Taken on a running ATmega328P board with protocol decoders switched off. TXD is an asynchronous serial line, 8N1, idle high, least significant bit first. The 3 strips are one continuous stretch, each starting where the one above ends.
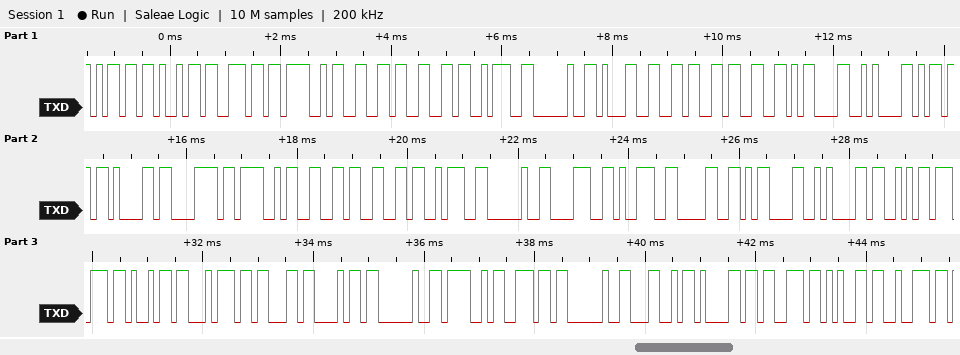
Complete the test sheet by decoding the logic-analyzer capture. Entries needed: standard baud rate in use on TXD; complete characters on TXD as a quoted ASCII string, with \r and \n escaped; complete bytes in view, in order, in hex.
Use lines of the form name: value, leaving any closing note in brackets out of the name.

standard baud rate in use on TXD: 9600 baud
complete characters on TXD as a quoted ASCII string, with \r and \n escaped: "minOff: 163\r\nmaxOff: 890\r\nSwitch On Laser"
complete bytes in view, in order, in hex: 0x6D 0x69 0x6E 0x4F 0x66 0x66 0x3A 0x20 0x31 0x36 0x33 0x0D 0x0A 0x6D 0x61 0x78 0x4F 0x66 0x66 0x3A 0x20 0x38 0x39 0x30 0x0D 0x0A 0x53 0x77 0x69 0x74 0x63 0x68 0x20 0x4F 0x6E 0x20 0x4C 0x61 0x73 0x65 0x72
